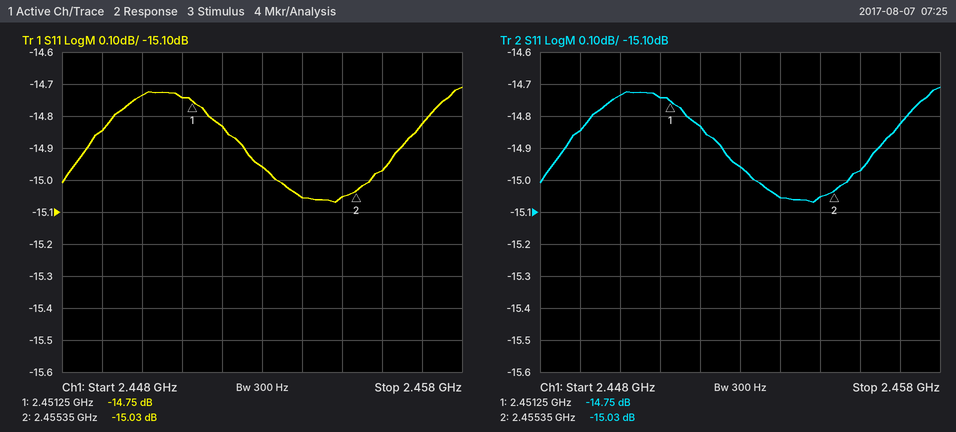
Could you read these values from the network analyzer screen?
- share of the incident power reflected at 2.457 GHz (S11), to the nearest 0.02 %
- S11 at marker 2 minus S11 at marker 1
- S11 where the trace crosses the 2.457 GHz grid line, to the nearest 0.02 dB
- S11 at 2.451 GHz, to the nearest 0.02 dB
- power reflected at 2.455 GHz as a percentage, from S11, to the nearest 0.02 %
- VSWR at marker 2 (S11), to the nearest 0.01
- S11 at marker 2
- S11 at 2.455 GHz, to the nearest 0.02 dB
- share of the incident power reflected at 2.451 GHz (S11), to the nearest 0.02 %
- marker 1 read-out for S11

3.30 %
-0.28 dB
-14.82 dB
-14.74 dB
3.12 %
1.43
-15.03 dB
-15.06 dB
3.36 %
-14.75 dB
